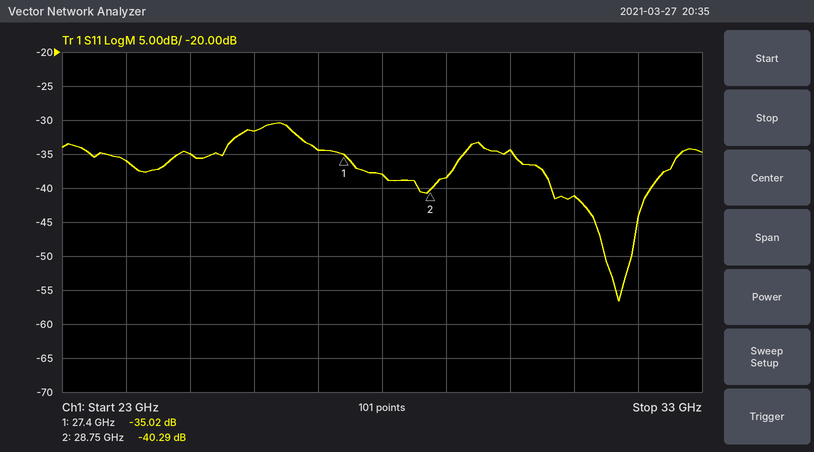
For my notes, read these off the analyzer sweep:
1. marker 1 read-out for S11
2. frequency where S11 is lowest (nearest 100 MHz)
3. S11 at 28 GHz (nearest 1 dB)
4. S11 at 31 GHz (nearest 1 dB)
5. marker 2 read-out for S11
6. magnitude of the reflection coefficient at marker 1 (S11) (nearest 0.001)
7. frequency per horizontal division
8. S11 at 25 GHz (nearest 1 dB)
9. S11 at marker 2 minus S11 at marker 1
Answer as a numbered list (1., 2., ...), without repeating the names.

1. -35.02 dB
2. 31.7 GHz
3. -38 dB
4. -41 dB
5. -40.29 dB
6. 0.018
7. 1 GHz
8. -35 dB
9. -5.27 dB
